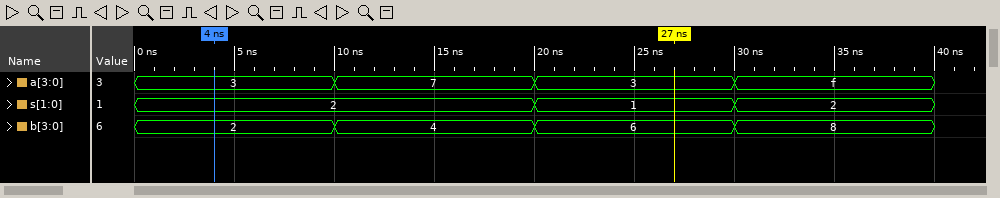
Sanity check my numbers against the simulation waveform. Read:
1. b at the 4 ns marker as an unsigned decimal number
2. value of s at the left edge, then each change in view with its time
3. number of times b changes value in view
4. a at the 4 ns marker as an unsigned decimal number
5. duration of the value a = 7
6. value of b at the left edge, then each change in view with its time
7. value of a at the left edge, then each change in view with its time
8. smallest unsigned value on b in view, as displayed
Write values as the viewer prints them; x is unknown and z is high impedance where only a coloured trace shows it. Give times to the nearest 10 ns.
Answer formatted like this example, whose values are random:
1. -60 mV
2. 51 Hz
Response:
1. 2
2. 2, 1 at 20 ns, 2 at 30 ns
3. 3
4. 3
5. 10 ns
6. 2, 4 at 10 ns, 6 at 20 ns, 8 at 30 ns
7. 3, 7 at 10 ns, 3 at 20 ns, f at 30 ns
8. 2
